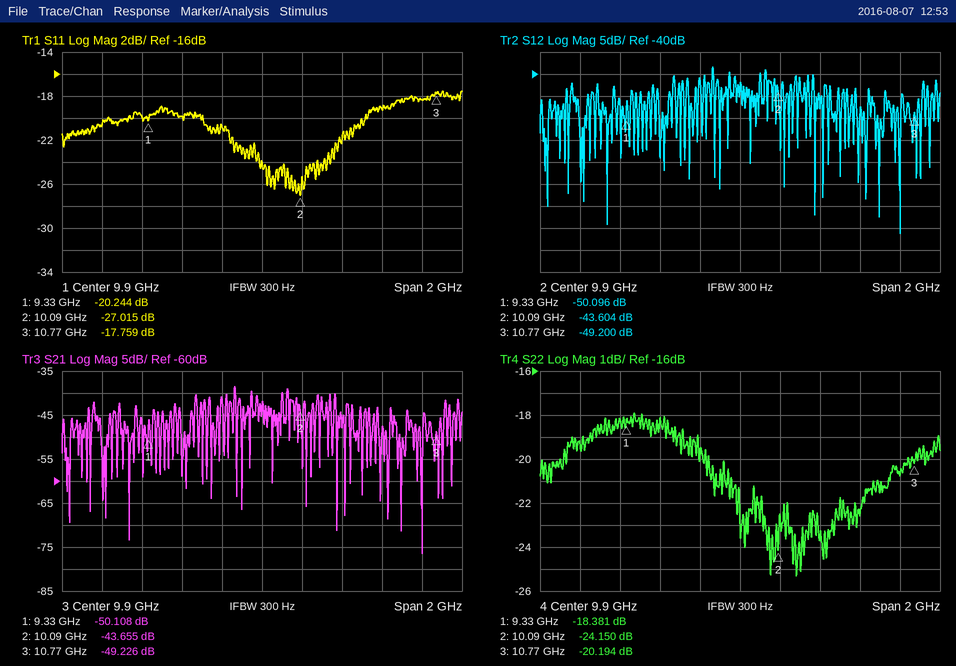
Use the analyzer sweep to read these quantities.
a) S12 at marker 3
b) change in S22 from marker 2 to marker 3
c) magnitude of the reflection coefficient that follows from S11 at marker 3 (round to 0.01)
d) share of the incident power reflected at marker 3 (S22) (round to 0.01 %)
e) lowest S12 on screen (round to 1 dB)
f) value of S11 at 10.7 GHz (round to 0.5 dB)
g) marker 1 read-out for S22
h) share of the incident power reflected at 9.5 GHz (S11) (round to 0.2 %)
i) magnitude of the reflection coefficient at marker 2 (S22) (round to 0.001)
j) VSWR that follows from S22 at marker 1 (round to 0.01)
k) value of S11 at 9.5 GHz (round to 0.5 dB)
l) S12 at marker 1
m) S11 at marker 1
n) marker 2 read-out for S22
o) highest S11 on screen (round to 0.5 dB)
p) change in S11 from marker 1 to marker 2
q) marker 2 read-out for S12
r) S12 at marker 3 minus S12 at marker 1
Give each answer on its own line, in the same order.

-49.200 dB
3.956 dB
0.13
0.96 %
-76 dB
-18.5 dB
-18.381 dB
1.0 %
0.062
1.27
-20.0 dB
-50.096 dB
-20.244 dB
-24.150 dB
-17.5 dB
-6.771 dB
-43.604 dB
0.896 dB
